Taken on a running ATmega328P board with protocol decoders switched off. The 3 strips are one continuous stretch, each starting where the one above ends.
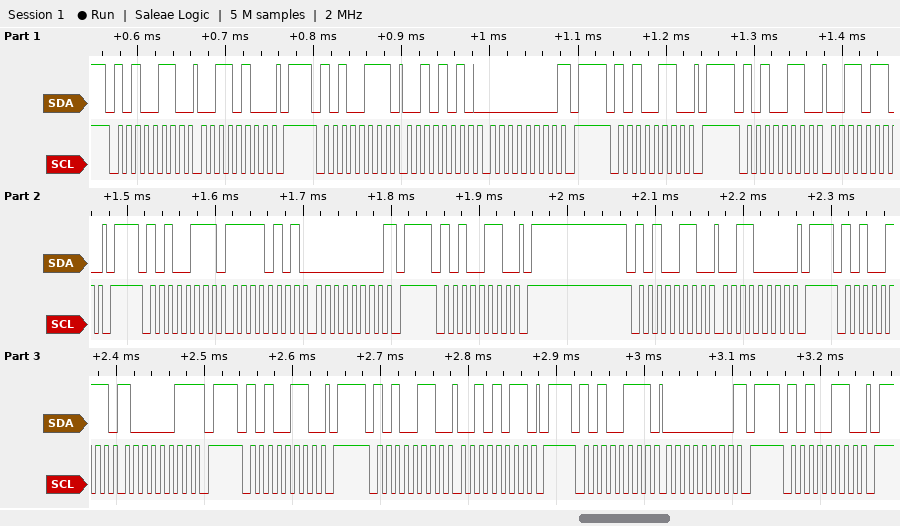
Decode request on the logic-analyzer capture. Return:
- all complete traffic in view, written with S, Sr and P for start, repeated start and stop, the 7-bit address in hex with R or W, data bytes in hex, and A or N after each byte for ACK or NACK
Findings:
S 53W A 34 A P S 53R A 2A A 00 N P S 53W A P S 53W A 36 A P S 53R A F5 A 00 N P S 53W A P S 53W A 30 A P S 53R A 83 N P S 53W A P S 53W A 2B A P S 53R A 00 N P S 53W A P
